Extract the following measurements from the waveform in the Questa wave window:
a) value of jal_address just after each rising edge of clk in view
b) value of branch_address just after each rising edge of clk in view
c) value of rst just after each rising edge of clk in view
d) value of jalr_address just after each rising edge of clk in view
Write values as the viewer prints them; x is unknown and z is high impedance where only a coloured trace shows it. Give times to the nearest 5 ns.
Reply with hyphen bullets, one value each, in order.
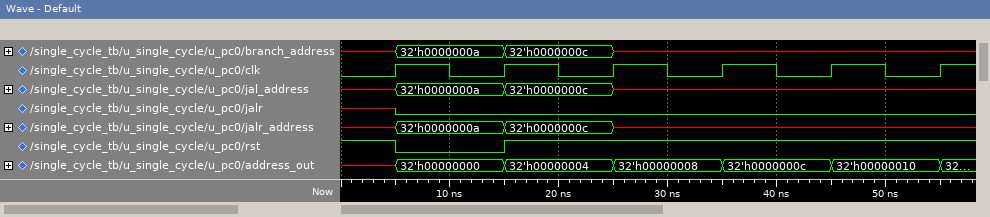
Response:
- 32'h0000000a, 32'h0000000c, x, x, x, x
- 32'h0000000a, 32'h0000000c, x, x, x, x
- 0 1 1 1 1 1
- 32'h0000000a, 32'h0000000c, x, x, x, x
